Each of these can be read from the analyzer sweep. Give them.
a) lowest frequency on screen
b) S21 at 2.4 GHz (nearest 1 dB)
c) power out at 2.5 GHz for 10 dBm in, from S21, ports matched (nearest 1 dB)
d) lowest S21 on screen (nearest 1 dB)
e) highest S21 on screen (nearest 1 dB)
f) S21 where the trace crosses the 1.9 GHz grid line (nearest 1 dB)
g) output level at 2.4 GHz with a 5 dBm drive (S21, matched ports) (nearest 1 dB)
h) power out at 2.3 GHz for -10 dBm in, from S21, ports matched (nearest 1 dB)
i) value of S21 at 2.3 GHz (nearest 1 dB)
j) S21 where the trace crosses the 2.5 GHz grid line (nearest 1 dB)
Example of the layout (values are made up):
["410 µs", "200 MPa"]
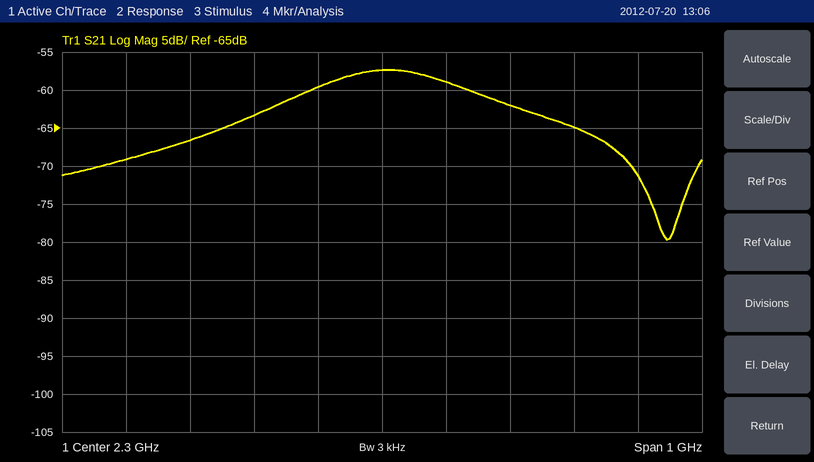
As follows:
["1.8 GHz", "-59 dB", "-52 dBm", "-80 dB", "-57 dB", "-69 dB", "-54 dBm", "-67 dBm", "-57 dB", "-62 dB"]
